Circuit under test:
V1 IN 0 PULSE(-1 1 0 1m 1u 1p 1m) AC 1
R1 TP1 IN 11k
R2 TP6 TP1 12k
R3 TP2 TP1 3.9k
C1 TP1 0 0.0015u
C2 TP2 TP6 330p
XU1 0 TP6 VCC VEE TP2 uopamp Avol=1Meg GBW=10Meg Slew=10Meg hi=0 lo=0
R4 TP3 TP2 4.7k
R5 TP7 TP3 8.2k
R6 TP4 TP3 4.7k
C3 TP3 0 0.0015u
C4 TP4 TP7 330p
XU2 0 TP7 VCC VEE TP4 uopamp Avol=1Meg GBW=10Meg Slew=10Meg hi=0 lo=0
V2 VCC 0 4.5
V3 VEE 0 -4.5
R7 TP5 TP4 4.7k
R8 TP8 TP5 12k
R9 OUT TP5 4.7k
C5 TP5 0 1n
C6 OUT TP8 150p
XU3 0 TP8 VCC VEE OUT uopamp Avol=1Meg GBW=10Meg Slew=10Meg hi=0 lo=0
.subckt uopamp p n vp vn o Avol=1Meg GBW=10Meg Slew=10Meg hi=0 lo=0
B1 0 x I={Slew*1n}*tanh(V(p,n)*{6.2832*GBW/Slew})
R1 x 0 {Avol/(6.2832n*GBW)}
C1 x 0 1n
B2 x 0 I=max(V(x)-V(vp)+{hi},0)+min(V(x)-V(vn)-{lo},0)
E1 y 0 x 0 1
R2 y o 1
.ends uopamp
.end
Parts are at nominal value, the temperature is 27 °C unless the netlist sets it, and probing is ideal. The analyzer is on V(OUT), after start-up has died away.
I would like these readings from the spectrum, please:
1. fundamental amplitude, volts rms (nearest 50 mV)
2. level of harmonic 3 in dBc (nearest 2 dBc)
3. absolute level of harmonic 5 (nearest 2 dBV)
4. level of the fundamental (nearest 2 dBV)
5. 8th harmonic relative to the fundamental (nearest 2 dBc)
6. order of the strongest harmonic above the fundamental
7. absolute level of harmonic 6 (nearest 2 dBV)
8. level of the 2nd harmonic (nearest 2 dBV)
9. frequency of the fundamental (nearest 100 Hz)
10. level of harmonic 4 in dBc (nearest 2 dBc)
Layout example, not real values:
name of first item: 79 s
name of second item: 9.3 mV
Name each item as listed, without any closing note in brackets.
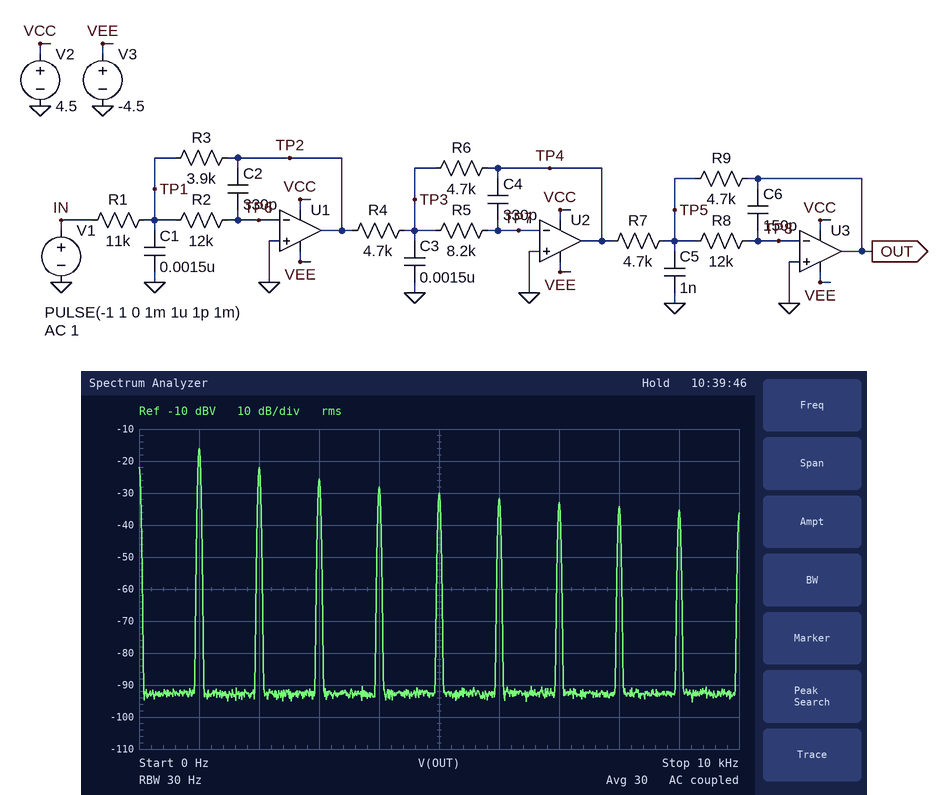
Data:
fundamental amplitude, volts rms: 150 mV
level of harmonic 3 in dBc: -10 dBc
absolute level of harmonic 5: -30 dBV
level of the fundamental: -16 dBV
8th harmonic relative to the fundamental: -18 dBc
order of the strongest harmonic above the fundamental: 2
absolute level of harmonic 6: -32 dBV
level of the 2nd harmonic: -22 dBV
frequency of the fundamental: 1.0 kHz
level of harmonic 4 in dBc: -12 dBc
